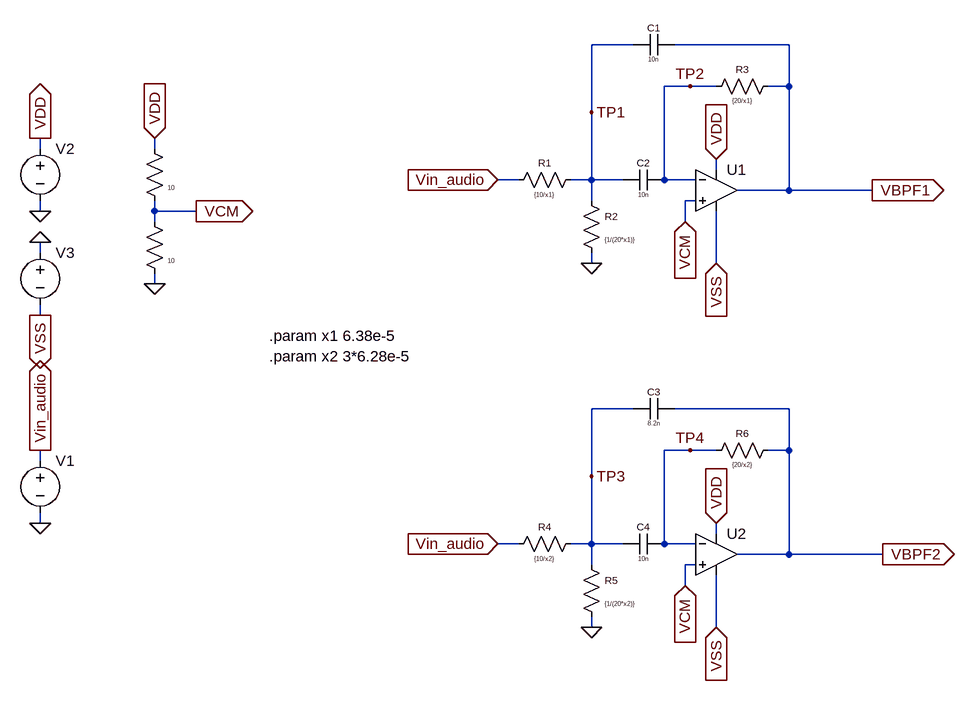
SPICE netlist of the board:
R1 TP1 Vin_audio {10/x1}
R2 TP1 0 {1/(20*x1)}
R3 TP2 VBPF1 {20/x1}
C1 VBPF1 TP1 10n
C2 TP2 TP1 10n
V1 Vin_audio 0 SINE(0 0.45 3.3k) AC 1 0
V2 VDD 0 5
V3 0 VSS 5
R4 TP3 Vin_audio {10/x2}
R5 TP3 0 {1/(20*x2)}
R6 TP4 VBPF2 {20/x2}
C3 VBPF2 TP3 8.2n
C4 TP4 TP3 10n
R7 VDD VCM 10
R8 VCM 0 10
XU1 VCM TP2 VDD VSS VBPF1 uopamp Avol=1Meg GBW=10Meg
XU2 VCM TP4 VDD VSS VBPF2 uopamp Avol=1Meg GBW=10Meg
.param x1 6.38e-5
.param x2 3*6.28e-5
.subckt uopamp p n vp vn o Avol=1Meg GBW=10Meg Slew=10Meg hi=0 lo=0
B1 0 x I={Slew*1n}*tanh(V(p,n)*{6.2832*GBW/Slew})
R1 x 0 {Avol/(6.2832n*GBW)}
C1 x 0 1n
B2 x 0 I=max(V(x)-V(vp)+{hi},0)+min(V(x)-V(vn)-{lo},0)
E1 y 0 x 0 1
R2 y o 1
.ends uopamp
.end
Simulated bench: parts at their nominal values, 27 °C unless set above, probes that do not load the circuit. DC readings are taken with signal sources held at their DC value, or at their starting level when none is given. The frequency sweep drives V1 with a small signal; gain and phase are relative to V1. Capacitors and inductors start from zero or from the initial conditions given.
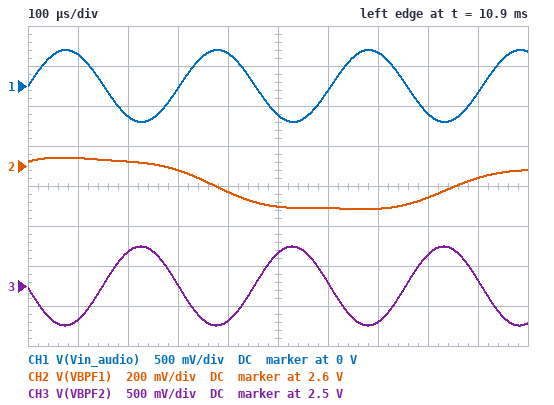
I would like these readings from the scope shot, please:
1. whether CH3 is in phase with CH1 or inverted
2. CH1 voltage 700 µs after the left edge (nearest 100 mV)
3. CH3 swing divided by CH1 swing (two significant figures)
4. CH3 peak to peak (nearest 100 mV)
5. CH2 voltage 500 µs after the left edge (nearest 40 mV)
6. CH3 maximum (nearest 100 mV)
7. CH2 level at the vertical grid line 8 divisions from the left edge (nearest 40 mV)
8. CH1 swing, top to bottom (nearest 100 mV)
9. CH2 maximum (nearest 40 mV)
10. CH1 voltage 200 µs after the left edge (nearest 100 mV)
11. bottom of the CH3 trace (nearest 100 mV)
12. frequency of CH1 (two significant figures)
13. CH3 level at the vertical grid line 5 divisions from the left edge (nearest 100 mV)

inverted
400 mV
1.1
1.0 V
2.40 V
3.0 V
2.44 V
900 mV
2.64 V
-400 mV
2.0 V
3.3 kHz
2.9 V
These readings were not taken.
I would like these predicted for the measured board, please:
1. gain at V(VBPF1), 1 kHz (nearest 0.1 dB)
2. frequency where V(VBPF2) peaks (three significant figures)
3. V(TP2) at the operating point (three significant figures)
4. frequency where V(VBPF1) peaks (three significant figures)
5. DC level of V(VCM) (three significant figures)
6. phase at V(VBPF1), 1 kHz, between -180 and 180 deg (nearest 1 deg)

-0.5 dB
3.31 kHz
2.50 V
1.02 kHz
2.50 V
-161 deg
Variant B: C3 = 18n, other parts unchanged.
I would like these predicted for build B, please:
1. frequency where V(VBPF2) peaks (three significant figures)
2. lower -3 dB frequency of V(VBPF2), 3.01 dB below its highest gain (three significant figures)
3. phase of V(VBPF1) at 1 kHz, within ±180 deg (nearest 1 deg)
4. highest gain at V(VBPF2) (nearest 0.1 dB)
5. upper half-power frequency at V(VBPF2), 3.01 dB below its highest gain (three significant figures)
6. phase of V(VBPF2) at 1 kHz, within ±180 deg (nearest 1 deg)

2.24 kHz
2.12 kHz
-161 deg
-2.9 dB
2.36 kHz
-93 deg
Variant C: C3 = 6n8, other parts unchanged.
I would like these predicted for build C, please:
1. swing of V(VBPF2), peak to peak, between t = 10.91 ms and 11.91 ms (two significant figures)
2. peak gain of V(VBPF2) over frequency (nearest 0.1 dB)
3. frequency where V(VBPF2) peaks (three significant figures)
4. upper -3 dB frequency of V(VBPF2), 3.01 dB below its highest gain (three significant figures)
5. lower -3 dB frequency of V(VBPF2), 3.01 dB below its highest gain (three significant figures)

500 mV
1.5 dB
3.63 kHz
3.82 kHz
3.45 kHz
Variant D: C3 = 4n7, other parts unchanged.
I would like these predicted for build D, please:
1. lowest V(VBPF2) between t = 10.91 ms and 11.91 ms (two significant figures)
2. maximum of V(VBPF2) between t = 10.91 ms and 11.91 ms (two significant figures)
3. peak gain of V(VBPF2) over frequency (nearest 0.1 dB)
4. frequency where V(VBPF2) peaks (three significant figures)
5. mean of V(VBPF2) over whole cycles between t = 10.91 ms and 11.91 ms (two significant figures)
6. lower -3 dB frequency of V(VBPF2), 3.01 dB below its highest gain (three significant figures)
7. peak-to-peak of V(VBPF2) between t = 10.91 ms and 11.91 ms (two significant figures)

2.4 V
2.6 V
2.7 dB
4.36 kHz
2.5 V
4.13 kHz
230 mV
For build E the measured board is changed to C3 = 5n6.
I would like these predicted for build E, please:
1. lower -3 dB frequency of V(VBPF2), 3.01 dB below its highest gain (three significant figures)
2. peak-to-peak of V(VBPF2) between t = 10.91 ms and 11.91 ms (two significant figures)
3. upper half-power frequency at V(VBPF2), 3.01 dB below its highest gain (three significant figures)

3.79 kHz
300 mV
4.21 kHz
